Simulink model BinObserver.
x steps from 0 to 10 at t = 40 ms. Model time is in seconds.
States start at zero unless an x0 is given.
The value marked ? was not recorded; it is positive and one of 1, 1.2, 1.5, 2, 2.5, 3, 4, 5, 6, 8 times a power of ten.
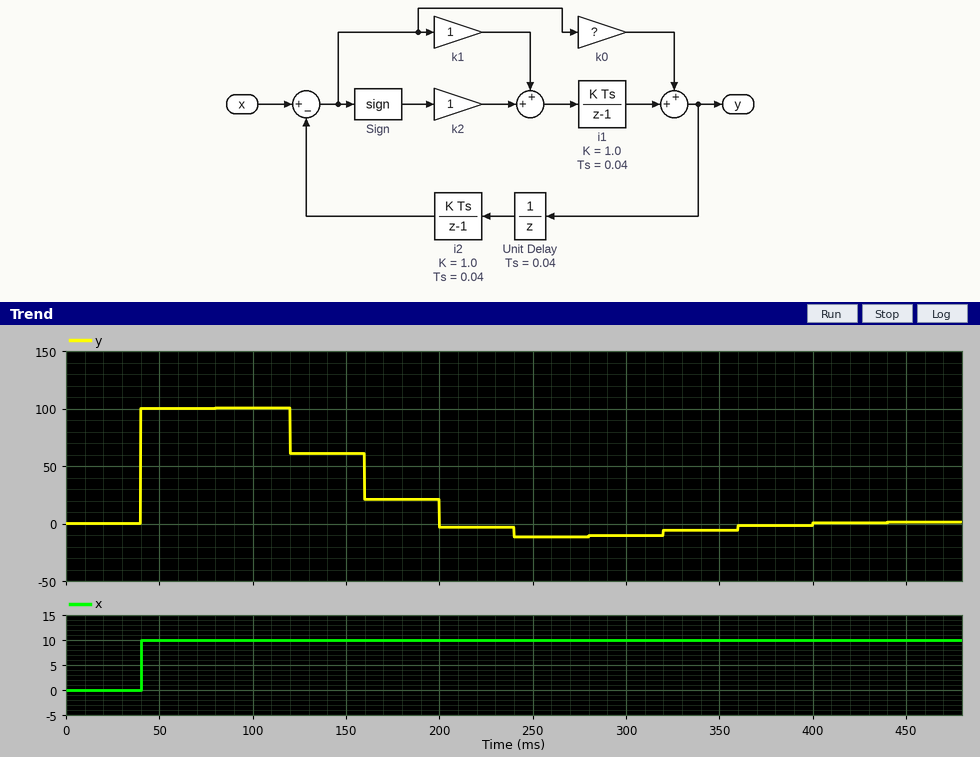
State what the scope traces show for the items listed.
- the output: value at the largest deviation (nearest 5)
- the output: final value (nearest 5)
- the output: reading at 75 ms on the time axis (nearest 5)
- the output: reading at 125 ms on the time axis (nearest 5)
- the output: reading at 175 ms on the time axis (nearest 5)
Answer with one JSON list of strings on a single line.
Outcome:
["100", "0", "100", "60", "20"]
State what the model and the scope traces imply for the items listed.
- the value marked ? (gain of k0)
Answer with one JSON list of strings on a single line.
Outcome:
["10"]
